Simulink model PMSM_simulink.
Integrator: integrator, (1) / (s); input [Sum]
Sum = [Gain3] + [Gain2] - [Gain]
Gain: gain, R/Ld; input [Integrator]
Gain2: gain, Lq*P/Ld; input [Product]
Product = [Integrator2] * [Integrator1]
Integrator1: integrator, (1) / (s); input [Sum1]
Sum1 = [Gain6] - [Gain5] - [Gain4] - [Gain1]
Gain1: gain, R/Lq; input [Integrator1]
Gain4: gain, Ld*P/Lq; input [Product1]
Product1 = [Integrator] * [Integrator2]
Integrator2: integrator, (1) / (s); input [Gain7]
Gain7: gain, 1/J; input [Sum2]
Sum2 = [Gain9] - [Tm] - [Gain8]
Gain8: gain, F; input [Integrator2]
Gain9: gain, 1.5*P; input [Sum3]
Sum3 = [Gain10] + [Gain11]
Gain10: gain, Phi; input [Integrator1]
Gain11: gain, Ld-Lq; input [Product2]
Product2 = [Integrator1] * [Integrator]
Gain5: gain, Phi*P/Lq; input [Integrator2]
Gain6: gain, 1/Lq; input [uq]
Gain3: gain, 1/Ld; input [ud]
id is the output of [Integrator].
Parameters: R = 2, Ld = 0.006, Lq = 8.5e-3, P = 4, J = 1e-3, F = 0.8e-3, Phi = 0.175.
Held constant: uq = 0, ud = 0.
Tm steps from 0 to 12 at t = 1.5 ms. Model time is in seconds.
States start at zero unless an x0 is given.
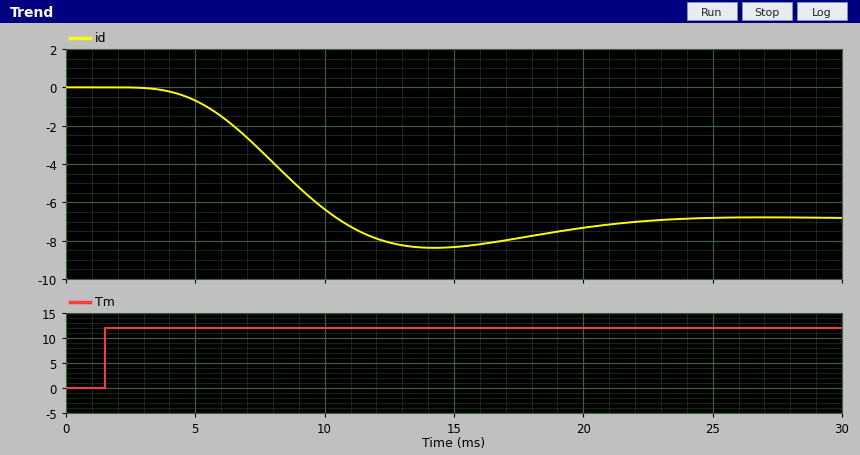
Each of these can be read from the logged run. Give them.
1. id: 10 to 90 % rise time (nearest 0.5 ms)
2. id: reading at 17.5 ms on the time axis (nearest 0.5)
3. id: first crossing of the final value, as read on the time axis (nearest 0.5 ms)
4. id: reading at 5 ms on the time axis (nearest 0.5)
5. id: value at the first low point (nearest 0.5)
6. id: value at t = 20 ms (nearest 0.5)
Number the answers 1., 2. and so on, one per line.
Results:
1. 5.0 ms
2. -8.0
3. 10.5 ms
4. -0.5
5. -8.5
6. -7.5
